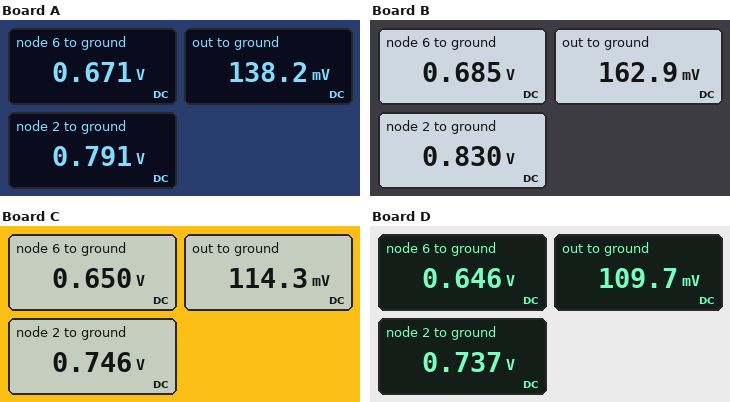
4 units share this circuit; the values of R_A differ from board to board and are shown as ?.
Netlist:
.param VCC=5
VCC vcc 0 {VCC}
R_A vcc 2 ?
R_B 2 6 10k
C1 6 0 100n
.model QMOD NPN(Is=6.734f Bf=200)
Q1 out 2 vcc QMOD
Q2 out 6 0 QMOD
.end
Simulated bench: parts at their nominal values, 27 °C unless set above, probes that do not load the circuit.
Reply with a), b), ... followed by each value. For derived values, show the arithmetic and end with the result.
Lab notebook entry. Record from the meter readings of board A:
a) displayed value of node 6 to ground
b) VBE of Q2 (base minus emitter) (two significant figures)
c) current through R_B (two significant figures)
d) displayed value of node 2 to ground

a) 0.671 V
b) 671 mV = 670 mV
c) (791 mV - 671 mV) / 10 kΩ = 12 µA
d) 0.791 V
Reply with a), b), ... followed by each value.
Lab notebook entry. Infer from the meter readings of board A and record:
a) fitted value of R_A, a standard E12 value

a) 6.8 kΩ
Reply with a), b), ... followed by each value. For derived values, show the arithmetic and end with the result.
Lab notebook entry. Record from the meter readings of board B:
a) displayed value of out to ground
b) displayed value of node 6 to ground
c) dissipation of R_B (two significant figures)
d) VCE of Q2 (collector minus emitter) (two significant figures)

a) 162.9 mV
b) 0.685 V
c) (830 mV - 685 mV)^2 / 10 kΩ = 2.1 µW
d) 162.9 mV = 160 mV
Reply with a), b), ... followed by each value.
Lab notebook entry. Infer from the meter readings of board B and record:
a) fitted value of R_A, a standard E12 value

a) 3.9 kΩ
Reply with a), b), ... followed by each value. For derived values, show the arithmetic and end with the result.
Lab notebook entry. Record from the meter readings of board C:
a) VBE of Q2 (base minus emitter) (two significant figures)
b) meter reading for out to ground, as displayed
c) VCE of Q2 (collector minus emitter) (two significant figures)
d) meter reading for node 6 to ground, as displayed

a) 650 mV = 650 mV
b) 114.3 mV
c) 114.3 mV = 110 mV
d) 0.650 V
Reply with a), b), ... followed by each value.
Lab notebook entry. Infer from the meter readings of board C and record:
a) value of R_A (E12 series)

a) 15 kΩ
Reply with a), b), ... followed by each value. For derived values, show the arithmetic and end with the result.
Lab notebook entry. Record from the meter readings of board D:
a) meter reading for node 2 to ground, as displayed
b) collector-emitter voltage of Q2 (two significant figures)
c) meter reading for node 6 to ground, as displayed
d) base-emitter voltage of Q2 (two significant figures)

a) 0.737 V
b) 109.7 mV = 110 mV
c) 0.646 V
d) 646 mV = 650 mV
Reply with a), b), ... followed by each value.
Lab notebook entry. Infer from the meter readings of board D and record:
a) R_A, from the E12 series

a) 18 kΩ
